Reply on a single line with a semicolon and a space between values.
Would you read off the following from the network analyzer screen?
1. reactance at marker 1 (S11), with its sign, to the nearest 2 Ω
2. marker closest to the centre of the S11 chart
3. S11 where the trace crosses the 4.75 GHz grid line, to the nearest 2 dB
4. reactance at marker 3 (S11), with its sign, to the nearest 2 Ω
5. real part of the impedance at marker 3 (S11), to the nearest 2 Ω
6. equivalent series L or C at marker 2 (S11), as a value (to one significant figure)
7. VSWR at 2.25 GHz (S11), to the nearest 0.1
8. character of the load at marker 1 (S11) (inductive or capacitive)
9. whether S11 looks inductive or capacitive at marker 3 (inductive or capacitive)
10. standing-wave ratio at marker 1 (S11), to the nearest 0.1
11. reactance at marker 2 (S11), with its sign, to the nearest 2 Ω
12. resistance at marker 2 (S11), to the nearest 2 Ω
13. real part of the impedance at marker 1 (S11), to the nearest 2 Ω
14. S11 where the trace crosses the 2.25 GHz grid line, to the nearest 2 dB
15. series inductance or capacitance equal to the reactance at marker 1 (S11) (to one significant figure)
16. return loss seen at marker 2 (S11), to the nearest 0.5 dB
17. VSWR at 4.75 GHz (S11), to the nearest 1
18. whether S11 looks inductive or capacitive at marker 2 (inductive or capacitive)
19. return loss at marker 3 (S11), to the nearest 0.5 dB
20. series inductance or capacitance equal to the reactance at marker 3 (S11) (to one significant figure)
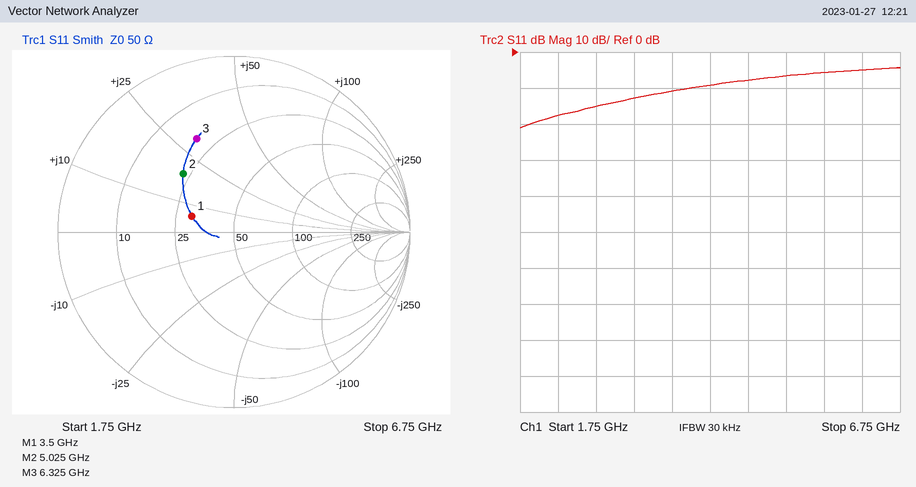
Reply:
+6 Ω; marker 1; -8 dB; +30 Ω; 20 Ω; 600 pH; 1.3; inductive; inductive; 1.7; +18 Ω; 22 Ω; 30 Ω; -18 dB; 300 pH; 7.0 dB; 2; inductive; 5.0 dB; 800 pH
